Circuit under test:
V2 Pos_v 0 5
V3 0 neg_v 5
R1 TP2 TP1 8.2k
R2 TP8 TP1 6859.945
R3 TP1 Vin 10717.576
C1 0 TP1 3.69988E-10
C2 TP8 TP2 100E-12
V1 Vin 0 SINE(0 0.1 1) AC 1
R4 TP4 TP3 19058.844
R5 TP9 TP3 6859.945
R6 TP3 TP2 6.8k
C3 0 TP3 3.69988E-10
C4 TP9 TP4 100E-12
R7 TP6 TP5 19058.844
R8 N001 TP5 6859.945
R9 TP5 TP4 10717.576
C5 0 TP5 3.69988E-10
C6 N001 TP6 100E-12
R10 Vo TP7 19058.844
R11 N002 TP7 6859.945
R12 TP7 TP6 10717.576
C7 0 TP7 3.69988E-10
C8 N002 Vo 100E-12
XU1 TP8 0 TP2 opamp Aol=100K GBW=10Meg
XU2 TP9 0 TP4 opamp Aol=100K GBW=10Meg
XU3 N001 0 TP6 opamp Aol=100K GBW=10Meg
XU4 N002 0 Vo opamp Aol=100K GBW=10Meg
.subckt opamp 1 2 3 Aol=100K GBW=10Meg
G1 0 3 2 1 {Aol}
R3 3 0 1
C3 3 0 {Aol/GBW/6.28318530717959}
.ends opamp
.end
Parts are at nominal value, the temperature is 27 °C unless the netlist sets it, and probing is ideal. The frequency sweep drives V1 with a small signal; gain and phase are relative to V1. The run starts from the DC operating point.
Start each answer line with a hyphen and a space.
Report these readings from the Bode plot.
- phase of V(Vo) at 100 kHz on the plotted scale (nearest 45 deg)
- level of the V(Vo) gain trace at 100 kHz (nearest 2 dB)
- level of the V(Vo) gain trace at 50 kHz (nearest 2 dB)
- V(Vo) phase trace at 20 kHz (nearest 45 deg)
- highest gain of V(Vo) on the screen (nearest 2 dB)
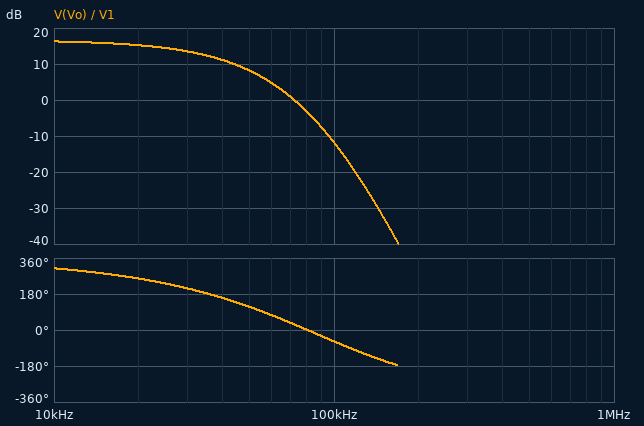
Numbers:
- -45 deg
- -12 dB
- 8 dB
- 270 deg
- 16 dB
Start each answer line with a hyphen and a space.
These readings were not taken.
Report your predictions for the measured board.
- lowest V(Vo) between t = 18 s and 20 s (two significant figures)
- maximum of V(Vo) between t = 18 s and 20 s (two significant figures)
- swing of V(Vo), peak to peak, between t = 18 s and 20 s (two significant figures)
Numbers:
- -680 mV
- 680 mV
- 1.4 V
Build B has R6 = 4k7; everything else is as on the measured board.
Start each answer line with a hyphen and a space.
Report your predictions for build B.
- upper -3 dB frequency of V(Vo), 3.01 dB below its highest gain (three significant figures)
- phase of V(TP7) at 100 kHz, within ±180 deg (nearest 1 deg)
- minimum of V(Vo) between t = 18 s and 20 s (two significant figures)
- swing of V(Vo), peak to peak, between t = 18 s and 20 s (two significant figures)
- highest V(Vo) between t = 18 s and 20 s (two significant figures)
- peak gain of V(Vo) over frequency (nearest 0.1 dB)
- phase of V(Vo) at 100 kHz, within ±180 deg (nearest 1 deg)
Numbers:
- 25.7 kHz
- -143 deg
- -980 mV
- 2.0 V
- 980 mV
- 19.8 dB
- -54 deg
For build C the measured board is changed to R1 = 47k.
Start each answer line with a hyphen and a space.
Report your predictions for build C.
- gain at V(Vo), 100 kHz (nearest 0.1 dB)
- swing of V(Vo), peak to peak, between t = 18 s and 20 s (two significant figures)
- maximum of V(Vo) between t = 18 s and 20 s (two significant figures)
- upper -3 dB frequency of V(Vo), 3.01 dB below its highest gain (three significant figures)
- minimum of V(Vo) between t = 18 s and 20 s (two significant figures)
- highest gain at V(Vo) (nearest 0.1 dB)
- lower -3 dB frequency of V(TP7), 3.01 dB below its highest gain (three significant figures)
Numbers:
- -10.7 dB
- 7.8 V
- 3.9 V
- 17.2 kHz
- -3.9 V
- 31.8 dB
- 10.6 kHz
